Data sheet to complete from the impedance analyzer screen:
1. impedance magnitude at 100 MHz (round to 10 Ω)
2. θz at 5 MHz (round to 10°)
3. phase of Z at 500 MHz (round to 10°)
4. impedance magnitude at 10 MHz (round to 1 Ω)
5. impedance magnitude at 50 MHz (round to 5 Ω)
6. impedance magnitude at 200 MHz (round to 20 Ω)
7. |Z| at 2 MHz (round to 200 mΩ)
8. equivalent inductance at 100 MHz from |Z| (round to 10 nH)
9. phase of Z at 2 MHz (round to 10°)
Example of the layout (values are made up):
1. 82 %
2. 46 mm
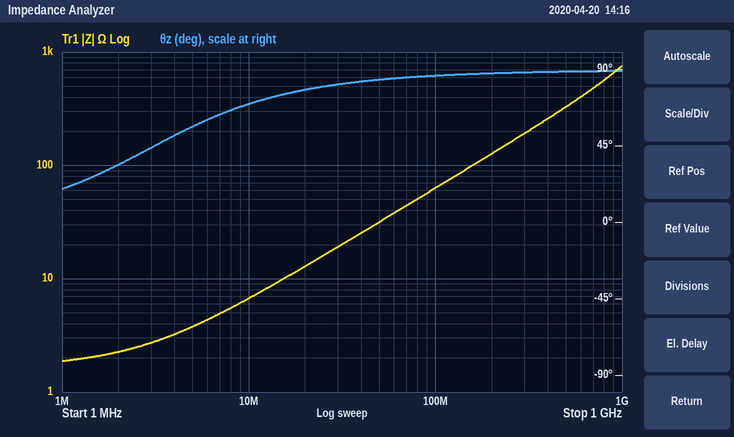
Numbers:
1. 60 Ω
2. 60°
3. 90°
4. 7 Ω
5. 30 Ω
6. 120 Ω
7. 2.2 Ω
8. 100 nH
9. 30°
